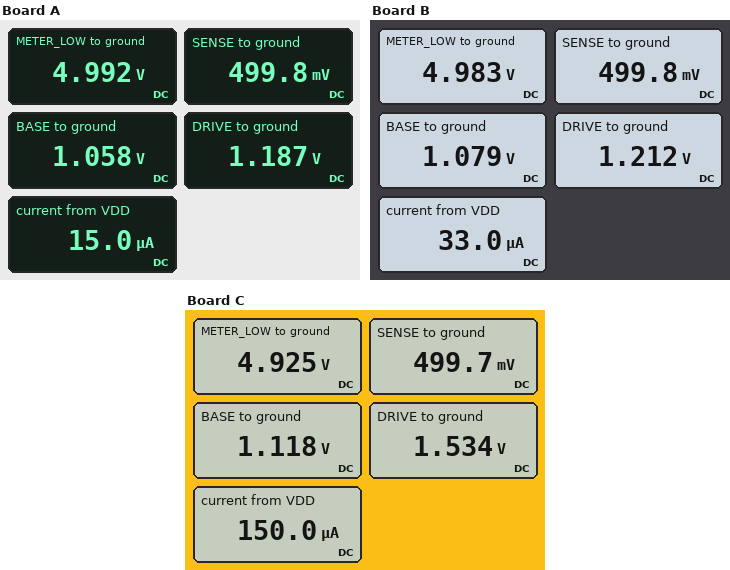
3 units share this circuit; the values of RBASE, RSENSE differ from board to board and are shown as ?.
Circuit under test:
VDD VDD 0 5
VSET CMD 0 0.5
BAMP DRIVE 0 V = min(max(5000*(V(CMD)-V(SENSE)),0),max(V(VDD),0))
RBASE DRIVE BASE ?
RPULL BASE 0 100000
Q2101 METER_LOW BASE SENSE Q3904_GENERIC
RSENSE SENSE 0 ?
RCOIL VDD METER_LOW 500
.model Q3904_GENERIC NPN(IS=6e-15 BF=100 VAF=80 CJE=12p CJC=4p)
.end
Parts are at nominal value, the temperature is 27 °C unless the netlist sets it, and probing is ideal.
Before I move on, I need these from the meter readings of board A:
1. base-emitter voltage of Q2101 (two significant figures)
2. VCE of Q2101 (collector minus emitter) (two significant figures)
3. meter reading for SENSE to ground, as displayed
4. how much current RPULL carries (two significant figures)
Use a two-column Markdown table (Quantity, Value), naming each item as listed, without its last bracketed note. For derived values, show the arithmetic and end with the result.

| Quantity | Value |
|---|---|
| base-emitter voltage of Q2101 | 1.058 V - 499.8 mV = 560 mV |
| VCE of Q2101 (collector minus emitter) | 4.992 V - 499.8 mV = 4.5 V |
| meter reading for SENSE to ground, as displayed | 499.8 mV |
| how much current RPULL carries | (1.058 V) / 100 kΩ = 11 µA |
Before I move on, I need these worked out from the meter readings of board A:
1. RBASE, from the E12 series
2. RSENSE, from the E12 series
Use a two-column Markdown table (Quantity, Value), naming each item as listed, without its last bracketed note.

| Quantity | Value |
|---|---|
| RBASE, from the E12 series | 12 kΩ |
| RSENSE, from the E12 series | 33 kΩ |
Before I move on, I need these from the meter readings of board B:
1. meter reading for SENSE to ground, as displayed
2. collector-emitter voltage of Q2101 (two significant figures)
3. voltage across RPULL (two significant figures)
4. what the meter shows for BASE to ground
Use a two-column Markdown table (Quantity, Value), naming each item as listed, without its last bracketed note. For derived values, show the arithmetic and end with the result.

| Quantity | Value |
|---|---|
| meter reading for SENSE to ground, as displayed | 499.8 mV |
| collector-emitter voltage of Q2101 | 4.983 V - 499.8 mV = 4.5 V |
| voltage across RPULL | 1.079 V = 1.1 V |
| what the meter shows for BASE to ground | 1.079 V |
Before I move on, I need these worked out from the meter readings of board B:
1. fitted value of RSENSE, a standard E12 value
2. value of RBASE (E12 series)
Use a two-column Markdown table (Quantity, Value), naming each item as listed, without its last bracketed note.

| Quantity | Value |
|---|---|
| fitted value of RSENSE, a standard E12 value | 15 kΩ |
| value of RBASE | 12 kΩ |
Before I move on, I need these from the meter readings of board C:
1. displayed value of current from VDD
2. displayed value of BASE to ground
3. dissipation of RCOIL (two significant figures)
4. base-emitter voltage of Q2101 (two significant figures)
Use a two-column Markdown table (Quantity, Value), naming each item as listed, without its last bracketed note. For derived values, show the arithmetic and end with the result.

| Quantity | Value |
|---|---|
| displayed value of current from VDD | 150.0 µA |
| displayed value of BASE to ground | 1.118 V |
| dissipation of RCOIL | (5 V - 4.925 V)^2 / 500 Ω = 11 µW |
| base-emitter voltage of Q2101 | 1.118 V - 499.7 mV = 620 mV |
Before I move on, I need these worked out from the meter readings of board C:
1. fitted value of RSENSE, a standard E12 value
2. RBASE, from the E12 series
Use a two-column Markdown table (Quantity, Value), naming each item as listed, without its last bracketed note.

| Quantity | Value |
|---|---|
| fitted value of RSENSE, a standard E12 value | 3.3 kΩ |
| RBASE, from the E12 series | 33 kΩ |
